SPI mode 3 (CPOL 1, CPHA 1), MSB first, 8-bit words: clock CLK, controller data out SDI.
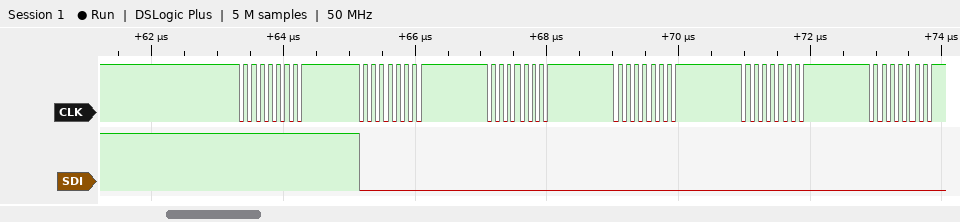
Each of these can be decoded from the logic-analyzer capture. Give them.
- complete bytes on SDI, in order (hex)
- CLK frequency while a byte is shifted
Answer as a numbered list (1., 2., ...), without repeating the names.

1. FF 00 00 00 00 00
2. 8 MHz
